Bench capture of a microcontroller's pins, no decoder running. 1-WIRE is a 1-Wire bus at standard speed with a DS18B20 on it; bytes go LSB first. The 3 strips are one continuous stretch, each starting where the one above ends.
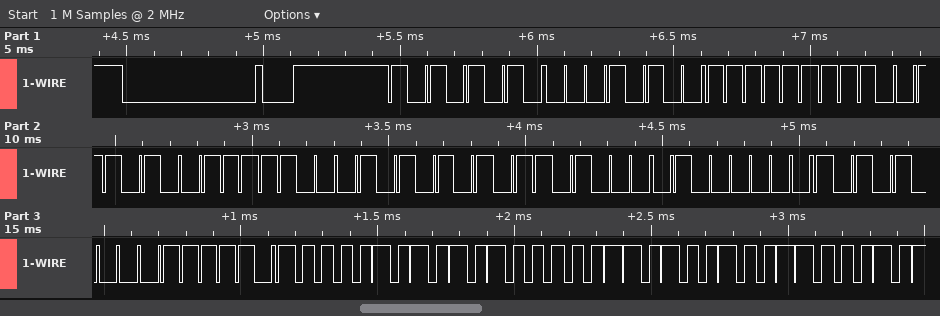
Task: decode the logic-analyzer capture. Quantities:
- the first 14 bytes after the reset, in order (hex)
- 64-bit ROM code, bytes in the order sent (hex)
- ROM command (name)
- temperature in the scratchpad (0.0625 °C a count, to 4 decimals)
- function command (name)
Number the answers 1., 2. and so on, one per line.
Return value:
1. 55 28 FF 59 3E AA 16 02 15 BE 50 05 4B 46
2. 28 FF 59 3E AA 16 02 15
3. Match ROM
4. 85.0000 °C
5. Read Scratchpad
